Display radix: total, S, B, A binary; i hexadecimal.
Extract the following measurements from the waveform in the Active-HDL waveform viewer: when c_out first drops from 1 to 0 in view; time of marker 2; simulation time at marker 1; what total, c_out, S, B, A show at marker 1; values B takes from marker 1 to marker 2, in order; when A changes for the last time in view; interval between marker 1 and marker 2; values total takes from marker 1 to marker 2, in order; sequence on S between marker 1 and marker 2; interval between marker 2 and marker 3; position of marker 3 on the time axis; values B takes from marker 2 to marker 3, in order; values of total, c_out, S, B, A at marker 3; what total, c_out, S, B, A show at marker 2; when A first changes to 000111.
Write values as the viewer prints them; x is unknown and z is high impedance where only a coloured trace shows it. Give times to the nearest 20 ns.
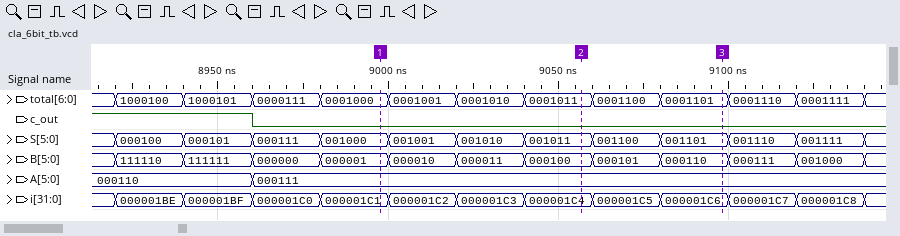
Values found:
8960 ns
9060 ns
9000 ns
total=0001000, c_out=0, S=001000, B=000001, A=000111
000001, 000010, 000011, 000100
8960 ns
60 ns
0001000, 0001001, 0001010, 0001011
001000, 001001, 001010, 001011
40 ns
9100 ns
000100, 000101, 000110
total=0001101, c_out=0, S=001101, B=000110, A=000111
total=0001011, c_out=0, S=001011, B=000100, A=000111
8960 ns
